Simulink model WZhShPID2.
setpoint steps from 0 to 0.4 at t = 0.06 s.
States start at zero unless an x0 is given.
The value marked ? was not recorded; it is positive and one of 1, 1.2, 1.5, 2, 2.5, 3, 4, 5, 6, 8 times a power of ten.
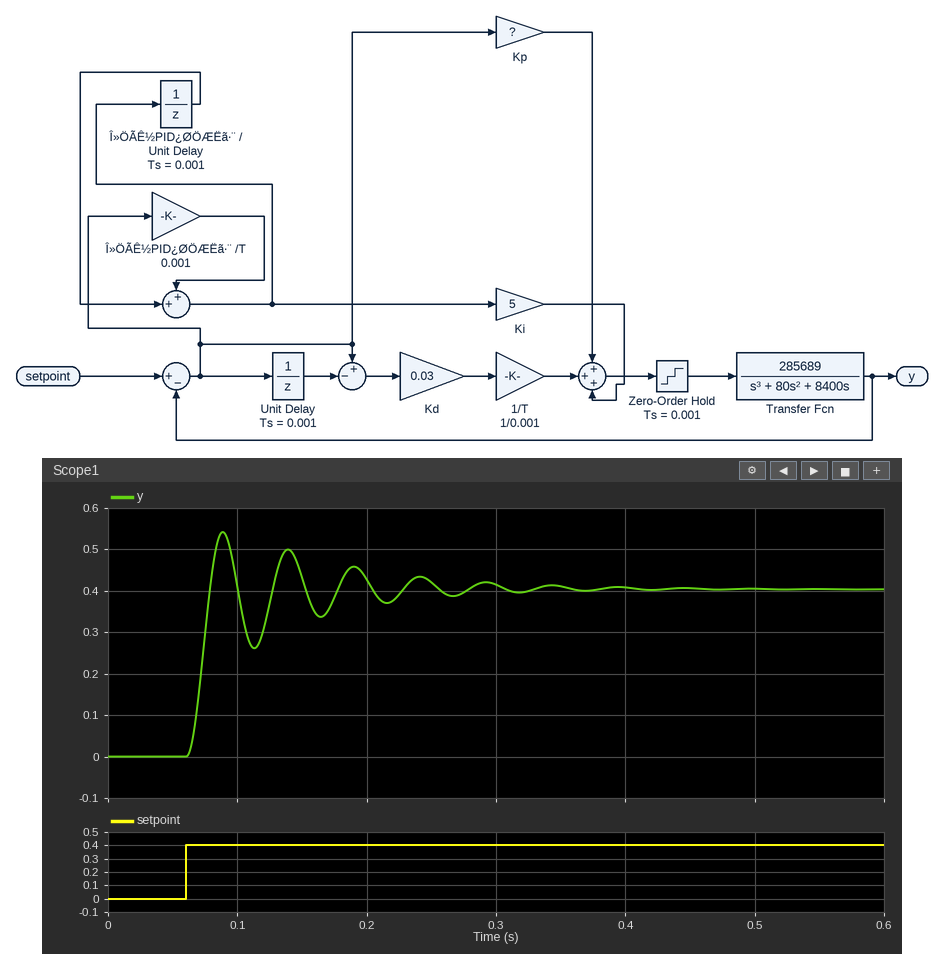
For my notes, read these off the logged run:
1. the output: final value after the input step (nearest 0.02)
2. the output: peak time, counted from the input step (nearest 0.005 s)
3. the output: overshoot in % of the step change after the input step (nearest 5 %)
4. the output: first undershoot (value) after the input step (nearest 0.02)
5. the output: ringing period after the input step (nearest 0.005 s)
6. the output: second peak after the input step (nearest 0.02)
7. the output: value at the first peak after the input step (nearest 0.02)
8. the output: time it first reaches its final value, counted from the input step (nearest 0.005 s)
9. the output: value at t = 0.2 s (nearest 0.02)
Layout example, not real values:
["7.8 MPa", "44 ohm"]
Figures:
["0.40", "0.030 s", "35 %", "0.26", "0.050 s", "0.50", "0.54", "0.020 s", "0.42"]
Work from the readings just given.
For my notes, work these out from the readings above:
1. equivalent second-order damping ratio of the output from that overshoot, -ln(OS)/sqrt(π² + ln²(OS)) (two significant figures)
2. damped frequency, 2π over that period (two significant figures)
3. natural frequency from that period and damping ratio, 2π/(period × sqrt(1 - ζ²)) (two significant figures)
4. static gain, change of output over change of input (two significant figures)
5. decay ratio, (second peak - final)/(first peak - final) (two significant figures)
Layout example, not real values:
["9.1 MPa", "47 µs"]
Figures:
["0.32", "130 rad/s", "130 rad/s", "1.0", "0.71"]
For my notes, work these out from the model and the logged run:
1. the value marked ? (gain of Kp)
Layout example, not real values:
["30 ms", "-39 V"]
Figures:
["2.5"]
